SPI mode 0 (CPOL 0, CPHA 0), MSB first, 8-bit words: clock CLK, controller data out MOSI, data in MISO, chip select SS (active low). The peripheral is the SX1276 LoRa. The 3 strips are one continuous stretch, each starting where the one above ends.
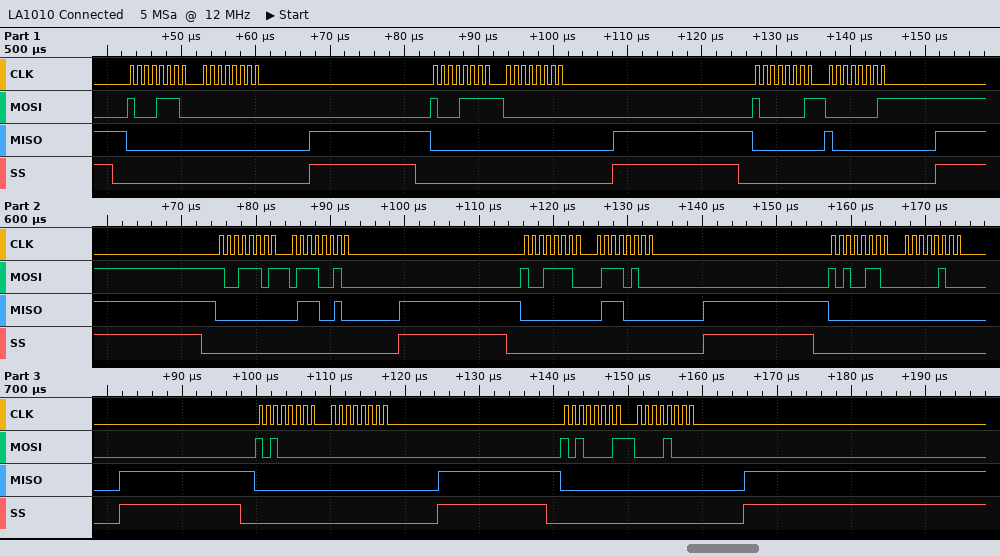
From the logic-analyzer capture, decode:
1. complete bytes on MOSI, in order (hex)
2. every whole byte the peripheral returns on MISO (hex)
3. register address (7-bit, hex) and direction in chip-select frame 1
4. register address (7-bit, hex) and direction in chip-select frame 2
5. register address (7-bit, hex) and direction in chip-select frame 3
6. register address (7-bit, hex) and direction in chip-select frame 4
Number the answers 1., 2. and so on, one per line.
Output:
1. 0x8E 0x00 0x8F 0x00 0x81 0x01 0x9D 0x72 0x9E 0x74 0xA6 0x04 0xA0 0x00 0xA1 0x08
2. 0x00 0x00 0x00 0x00 0x00 0x80 0x00 0x72 0x00 0x70 0x00 0x00 0x00 0x00 0x00 0x00
3. 0x0E write
4. 0x0F write
5. 0x01 write
6. 0x1D write
